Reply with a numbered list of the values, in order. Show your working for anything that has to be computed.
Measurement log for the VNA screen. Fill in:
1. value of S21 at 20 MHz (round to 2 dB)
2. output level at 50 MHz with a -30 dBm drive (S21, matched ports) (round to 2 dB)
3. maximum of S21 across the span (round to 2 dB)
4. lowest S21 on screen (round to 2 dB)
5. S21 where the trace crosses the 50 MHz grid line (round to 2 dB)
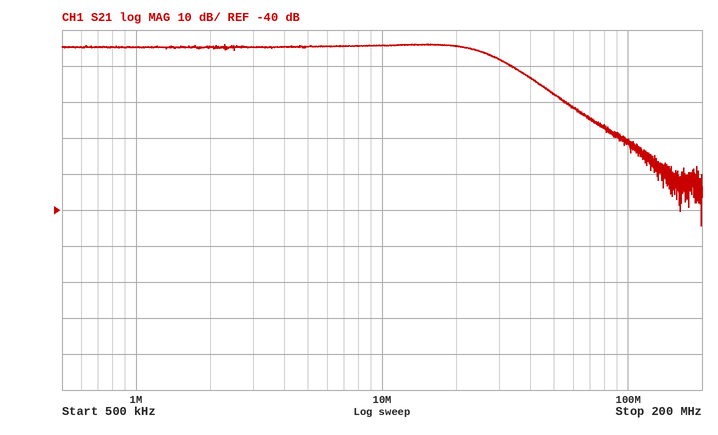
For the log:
1. 6 dB
2. -30 dBm + (-8 dB) = -38 dBm
3. 6 dB
4. -44 dB
5. -8 dB
